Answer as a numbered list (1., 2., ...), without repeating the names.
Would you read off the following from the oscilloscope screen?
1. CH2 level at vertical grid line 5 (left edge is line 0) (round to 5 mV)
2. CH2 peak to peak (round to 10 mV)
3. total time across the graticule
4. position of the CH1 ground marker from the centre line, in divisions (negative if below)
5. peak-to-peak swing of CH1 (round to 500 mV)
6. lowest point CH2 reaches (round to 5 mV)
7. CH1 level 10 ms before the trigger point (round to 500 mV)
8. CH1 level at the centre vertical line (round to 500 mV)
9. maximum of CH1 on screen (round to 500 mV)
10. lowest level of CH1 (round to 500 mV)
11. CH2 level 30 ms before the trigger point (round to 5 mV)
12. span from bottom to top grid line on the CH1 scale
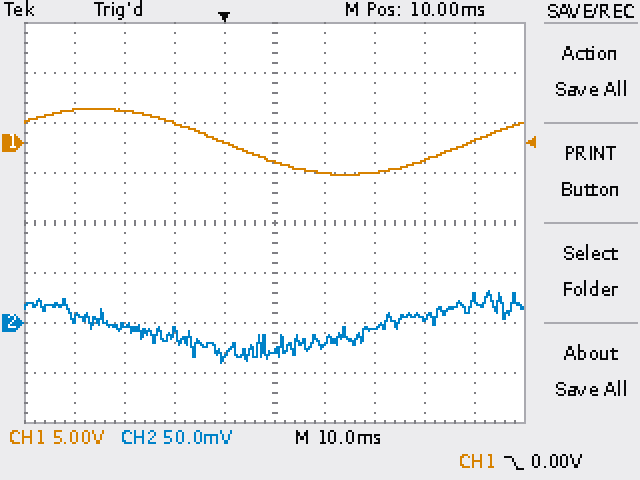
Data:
1. -25 mV
2. 70 mV
3. 100 ms
4. +1.6 div
5. 6.5 V
6. -40 mV
7. 2.0 V
8. -2.0 V
9. 3.5 V
10. -3.0 V
11. 5 mV
12. 40 V
